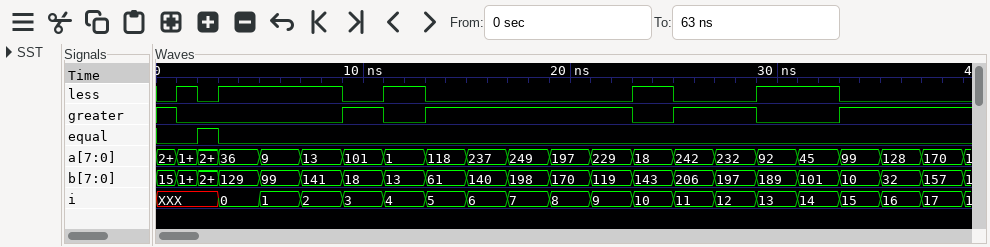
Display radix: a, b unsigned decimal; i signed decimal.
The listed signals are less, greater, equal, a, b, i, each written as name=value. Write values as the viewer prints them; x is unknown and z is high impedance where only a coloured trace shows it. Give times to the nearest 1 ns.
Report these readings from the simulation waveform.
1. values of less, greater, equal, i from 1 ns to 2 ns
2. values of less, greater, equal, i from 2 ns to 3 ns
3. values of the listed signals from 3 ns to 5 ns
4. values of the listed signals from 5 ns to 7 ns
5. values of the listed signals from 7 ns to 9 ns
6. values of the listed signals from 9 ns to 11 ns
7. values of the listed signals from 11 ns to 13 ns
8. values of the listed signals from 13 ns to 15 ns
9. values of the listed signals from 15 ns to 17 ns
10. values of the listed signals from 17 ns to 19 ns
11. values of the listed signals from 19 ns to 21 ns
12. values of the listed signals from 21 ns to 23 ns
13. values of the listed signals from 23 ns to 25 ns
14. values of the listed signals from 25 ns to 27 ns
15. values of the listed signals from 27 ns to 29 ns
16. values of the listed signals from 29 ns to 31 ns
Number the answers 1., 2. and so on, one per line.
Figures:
1. less=1, greater=0, equal=0, i=XXX
2. less=0, greater=0, equal=1, i=XXX
3. less=1, greater=0, equal=0, a=36, b=129, i=0
4. less=1, greater=0, equal=0, a=9, b=99, i=1
5. less=1, greater=0, equal=0, a=13, b=141, i=2
6. less=0, greater=1, equal=0, a=101, b=18, i=3
7. less=1, greater=0, equal=0, a=1, b=13, i=4
8. less=0, greater=1, equal=0, a=118, b=61, i=5
9. less=0, greater=1, equal=0, a=237, b=140, i=6
10. less=0, greater=1, equal=0, a=249, b=198, i=7
11. less=0, greater=1, equal=0, a=197, b=170, i=8
12. less=0, greater=1, equal=0, a=229, b=119, i=9
13. less=1, greater=0, equal=0, a=18, b=143, i=10
14. less=0, greater=1, equal=0, a=242, b=206, i=11
15. less=0, greater=1, equal=0, a=232, b=197, i=12
16. less=1, greater=0, equal=0, a=92, b=189, i=13
